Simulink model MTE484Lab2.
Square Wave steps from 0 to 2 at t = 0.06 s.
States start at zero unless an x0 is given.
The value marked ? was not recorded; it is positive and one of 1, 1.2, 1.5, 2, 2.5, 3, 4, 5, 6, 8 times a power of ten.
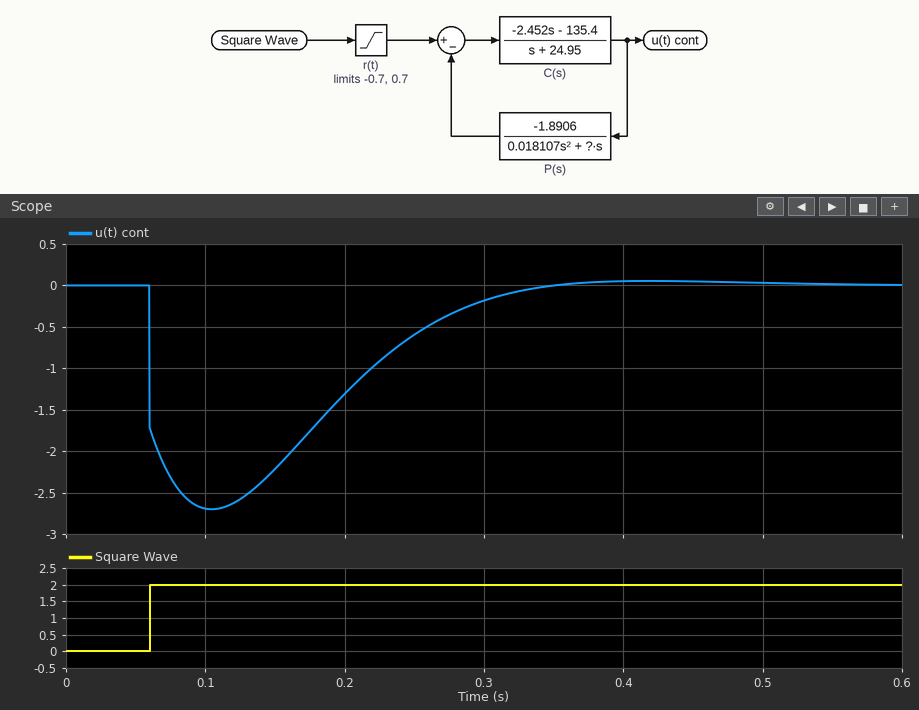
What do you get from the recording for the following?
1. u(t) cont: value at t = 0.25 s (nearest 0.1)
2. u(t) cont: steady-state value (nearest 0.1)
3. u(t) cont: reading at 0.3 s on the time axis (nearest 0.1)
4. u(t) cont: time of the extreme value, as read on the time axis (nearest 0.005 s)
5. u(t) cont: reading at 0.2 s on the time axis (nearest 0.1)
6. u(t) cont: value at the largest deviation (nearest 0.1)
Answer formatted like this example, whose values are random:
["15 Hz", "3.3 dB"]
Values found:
["-0.6", "0.0", "-0.2", "0.105 s", "-1.3", "-2.7"]
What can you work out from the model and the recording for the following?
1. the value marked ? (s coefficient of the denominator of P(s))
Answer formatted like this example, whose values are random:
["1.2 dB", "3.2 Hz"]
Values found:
["1"]
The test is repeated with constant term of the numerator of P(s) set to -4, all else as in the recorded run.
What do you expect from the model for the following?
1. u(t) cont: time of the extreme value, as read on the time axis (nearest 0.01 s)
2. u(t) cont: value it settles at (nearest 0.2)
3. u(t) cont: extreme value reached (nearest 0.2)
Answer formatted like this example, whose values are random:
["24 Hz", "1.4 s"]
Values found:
["0.09 s", "0.0", "-2.4"]
